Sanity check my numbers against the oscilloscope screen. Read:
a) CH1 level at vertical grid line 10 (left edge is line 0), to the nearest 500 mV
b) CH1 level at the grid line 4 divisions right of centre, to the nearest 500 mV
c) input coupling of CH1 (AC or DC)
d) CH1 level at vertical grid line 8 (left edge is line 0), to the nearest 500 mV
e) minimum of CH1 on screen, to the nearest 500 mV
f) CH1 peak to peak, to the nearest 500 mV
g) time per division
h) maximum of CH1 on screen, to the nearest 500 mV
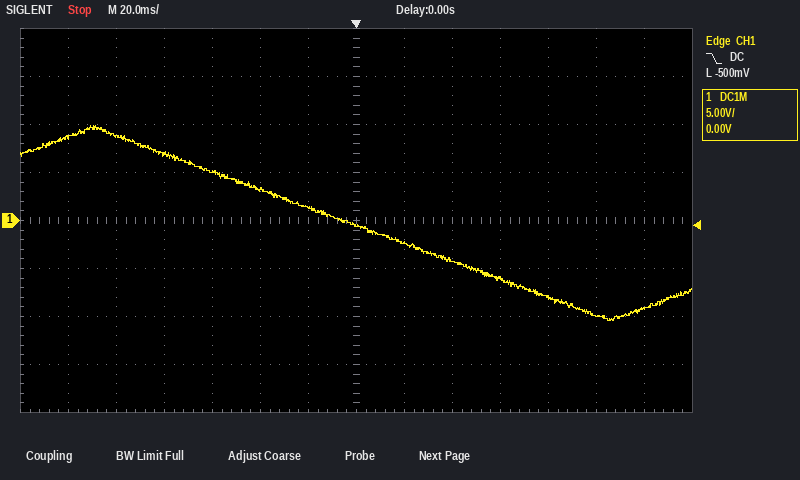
-6.0 V
-8.0 V
DC
-2.5 V
-10.5 V
20.5 V
20 ms
10.0 V
